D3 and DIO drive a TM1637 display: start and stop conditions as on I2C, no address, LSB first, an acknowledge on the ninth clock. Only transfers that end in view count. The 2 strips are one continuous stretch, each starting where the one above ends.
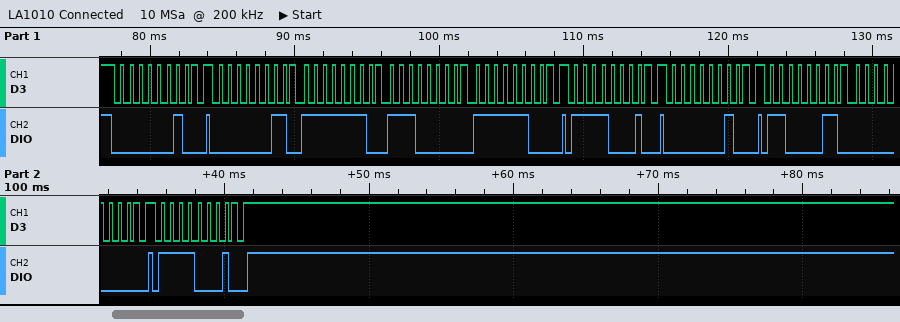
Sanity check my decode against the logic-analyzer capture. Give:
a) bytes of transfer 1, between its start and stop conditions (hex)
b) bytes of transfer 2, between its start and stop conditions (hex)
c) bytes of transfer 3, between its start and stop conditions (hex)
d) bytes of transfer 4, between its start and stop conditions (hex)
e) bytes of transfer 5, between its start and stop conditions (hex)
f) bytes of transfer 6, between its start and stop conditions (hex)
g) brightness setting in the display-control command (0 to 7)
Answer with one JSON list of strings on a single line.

["40", "C0 7F 07 3F", "8F", "40", "C3 00", "8F", "7"]
